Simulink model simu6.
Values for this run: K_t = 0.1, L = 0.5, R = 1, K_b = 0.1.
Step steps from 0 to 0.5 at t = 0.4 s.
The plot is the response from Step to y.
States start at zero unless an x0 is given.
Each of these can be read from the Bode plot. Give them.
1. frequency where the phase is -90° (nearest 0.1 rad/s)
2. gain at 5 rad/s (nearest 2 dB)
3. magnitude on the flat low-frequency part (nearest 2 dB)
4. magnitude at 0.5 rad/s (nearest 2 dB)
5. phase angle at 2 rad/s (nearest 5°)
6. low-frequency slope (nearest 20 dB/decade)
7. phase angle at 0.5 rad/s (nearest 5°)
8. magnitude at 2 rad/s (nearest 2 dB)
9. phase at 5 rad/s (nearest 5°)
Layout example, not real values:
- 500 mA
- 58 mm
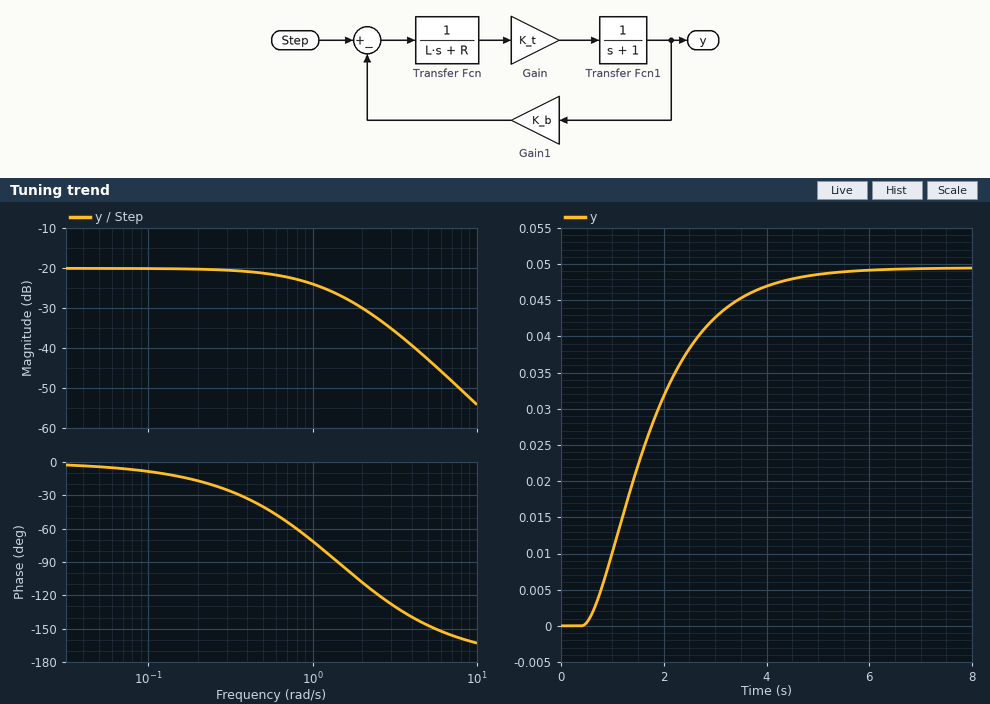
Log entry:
- 1.4 rad/s
- -42 dB
- -20 dB
- -22 dB
- -110°
- 0 dB/decade
- -40°
- -30 dB
- -145°
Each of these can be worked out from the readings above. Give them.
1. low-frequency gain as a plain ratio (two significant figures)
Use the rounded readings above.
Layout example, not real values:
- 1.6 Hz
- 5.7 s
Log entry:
- 0.10
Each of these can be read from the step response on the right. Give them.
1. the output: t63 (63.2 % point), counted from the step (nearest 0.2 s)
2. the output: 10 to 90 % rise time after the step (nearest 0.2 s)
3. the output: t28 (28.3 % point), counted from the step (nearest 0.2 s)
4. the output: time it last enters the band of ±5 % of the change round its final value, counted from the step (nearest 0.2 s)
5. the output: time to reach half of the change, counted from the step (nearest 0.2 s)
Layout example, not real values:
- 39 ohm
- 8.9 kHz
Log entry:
- 1.6 s
- 2.6 s
- 0.8 s
- 3.6 s
- 1.2 s
